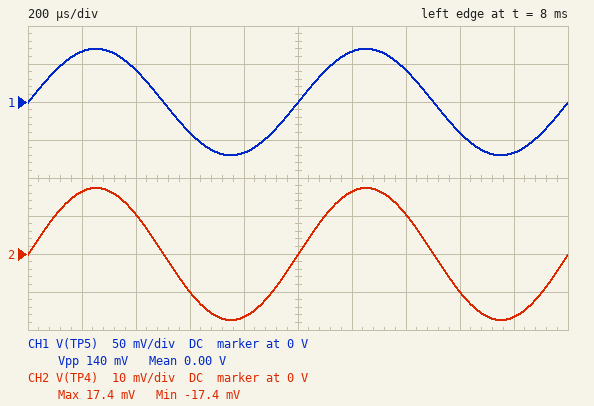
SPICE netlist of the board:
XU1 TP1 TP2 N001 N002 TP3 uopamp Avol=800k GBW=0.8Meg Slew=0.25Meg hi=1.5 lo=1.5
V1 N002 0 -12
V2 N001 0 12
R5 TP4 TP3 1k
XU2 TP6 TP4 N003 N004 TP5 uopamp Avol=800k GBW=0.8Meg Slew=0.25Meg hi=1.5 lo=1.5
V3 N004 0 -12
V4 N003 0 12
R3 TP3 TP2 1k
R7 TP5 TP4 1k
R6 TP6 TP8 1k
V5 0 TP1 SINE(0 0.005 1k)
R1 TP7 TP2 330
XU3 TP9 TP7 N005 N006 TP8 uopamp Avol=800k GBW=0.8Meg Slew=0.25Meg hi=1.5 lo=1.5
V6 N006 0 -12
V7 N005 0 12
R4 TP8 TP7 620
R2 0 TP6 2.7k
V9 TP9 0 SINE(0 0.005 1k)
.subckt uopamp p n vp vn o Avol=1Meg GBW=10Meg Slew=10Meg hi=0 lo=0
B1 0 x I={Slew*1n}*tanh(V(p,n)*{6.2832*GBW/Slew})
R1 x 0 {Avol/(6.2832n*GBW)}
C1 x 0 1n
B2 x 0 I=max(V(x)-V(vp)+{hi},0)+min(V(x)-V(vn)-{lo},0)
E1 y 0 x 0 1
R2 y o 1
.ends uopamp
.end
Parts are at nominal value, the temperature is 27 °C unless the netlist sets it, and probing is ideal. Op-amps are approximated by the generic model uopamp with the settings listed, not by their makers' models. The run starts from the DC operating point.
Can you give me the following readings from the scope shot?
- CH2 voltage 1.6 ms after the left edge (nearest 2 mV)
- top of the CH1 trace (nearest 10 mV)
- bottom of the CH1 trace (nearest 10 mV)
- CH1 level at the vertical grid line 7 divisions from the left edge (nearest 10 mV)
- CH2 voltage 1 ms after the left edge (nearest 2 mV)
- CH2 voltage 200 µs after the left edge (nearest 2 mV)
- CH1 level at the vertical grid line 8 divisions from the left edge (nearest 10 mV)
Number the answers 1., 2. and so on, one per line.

1. -10 mV
2. 70 mV
3. -70 mV
4. 40 mV
5. 0 V
6. 16 mV
7. -40 mV
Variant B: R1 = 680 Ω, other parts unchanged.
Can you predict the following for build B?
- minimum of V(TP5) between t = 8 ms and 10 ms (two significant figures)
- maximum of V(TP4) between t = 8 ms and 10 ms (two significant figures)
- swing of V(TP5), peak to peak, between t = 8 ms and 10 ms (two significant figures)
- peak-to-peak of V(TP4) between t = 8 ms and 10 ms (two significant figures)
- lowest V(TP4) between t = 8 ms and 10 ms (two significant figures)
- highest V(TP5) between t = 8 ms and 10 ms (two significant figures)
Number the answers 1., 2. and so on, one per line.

1. -40 mV
2. 10 mV
3. 81 mV
4. 21 mV
5. -10 mV
6. 40 mV
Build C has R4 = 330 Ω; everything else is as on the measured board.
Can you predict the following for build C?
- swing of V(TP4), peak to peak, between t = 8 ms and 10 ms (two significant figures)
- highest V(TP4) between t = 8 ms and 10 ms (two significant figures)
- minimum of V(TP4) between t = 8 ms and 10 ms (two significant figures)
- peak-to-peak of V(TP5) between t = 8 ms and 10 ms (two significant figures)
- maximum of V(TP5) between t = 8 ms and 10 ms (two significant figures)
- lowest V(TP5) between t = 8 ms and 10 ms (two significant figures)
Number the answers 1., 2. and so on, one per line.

1. 22 mV
2. 11 mV
3. -11 mV
4. 110 mV
5. 57 mV
6. -57 mV
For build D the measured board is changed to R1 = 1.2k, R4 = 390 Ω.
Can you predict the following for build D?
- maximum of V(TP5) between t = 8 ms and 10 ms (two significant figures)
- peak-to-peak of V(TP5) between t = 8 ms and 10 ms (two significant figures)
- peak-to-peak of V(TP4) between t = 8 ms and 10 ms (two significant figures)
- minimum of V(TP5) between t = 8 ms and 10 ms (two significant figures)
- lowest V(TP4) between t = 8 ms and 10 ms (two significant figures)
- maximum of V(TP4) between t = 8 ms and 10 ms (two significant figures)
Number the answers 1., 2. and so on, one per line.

1. 25 mV
2. 51 mV
3. 12 mV
4. -25 mV
5. -6.0 mV
6. 6.0 mV
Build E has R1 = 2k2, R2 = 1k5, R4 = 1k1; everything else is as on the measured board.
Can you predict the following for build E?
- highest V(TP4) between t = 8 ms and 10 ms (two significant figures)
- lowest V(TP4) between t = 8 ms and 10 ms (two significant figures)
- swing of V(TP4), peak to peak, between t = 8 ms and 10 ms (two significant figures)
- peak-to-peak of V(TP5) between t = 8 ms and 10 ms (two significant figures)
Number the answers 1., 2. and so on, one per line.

1. 6.0 mV
2. -6.0 mV
3. 12 mV
4. 43 mV
